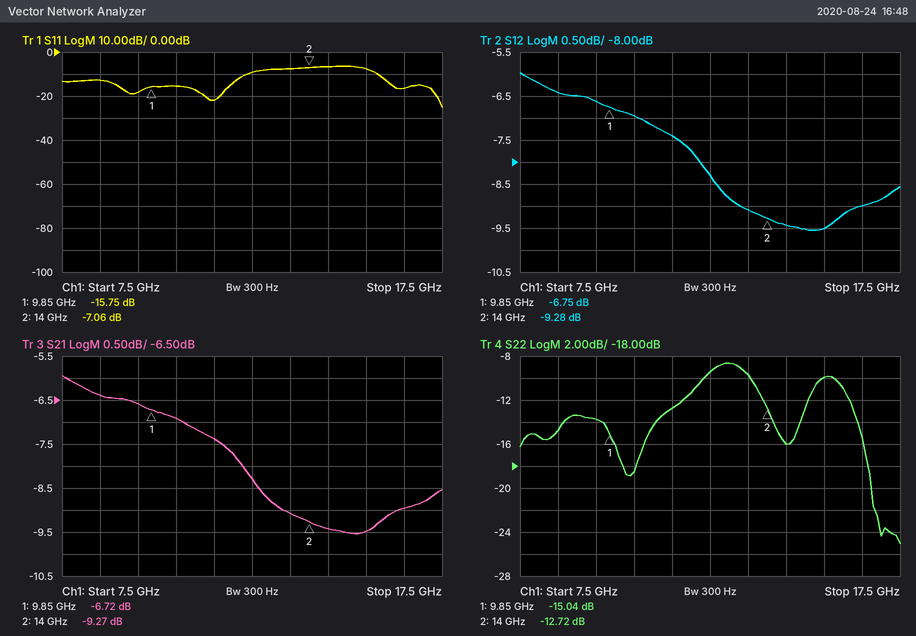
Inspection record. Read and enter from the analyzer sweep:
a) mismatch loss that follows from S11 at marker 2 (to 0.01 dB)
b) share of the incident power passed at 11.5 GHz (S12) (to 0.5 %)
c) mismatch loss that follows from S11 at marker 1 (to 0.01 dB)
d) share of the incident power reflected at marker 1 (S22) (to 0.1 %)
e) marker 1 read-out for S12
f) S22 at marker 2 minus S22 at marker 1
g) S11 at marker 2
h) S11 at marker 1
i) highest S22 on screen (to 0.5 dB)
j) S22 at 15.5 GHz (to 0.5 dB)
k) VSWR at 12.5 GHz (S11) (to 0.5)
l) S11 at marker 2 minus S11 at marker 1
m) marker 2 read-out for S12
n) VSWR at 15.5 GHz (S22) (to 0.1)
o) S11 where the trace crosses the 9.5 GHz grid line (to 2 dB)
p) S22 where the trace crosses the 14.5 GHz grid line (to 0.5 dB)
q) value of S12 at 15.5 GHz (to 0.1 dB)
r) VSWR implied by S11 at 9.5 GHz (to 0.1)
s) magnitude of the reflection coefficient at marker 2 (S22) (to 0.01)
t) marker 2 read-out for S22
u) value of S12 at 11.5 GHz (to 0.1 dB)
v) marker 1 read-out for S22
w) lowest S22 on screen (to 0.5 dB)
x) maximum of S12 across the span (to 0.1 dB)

0.95 dB
18.0 %
0.12 dB
3.1 %
-6.75 dB
2.32 dB
-7.06 dB
-15.75 dB
-8.5 dB
-10.0 dB
2.0
8.69 dB
-9.28 dB
1.9
-18 dB
-16.0 dB
-9.5 dB
1.3
0.23
-12.72 dB
-7.4 dB
-15.04 dB
-25.0 dB
-6.0 dB
